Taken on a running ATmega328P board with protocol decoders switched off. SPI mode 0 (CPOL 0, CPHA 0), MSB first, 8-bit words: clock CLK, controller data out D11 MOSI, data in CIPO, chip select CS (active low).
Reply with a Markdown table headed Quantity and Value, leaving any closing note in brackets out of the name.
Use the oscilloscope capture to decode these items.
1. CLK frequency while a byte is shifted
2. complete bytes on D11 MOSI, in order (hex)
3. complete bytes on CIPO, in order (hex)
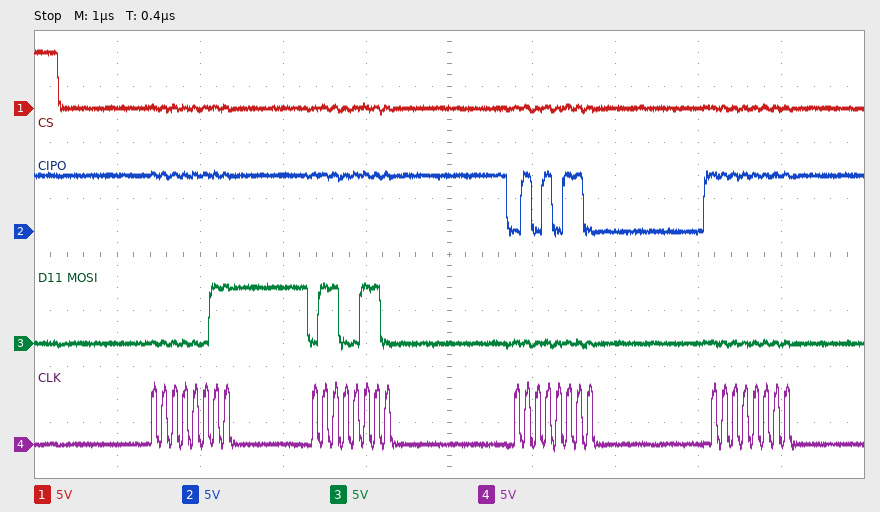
| Quantity | Value |
|---|---|
| CLK frequency while a byte is shifted | 8 MHz |
| complete bytes on D11 MOSI, in order | 03 66 00 00 |
| complete bytes on CIPO, in order | FF FF 56 FF |
